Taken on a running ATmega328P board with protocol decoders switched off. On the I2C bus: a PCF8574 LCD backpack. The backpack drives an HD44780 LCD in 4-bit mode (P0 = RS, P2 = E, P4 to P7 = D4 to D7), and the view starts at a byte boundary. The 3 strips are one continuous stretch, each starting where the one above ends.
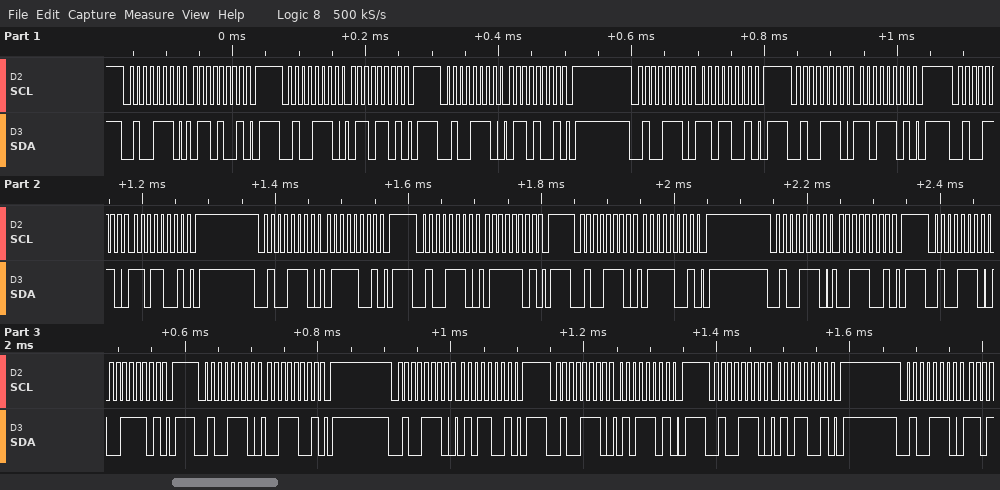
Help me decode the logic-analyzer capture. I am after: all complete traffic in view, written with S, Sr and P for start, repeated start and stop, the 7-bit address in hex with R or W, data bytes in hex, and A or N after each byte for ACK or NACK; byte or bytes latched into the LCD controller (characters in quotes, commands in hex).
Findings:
S 27W A 69 A P S 27W A 6D A P S 27W A 69 A P S 27W A D9 A P S 27W A DD A P S 27W A D9 A P S 27W A 79 A P S 27W A 7D A P S 27W A 79 A P S 27W A 39 A P S 27W A 3D A P S 27W A 39 A P S 27W A 59 A P S 27W A 5D A P S 27W A 59 A P S 27W A
'm' 's'
